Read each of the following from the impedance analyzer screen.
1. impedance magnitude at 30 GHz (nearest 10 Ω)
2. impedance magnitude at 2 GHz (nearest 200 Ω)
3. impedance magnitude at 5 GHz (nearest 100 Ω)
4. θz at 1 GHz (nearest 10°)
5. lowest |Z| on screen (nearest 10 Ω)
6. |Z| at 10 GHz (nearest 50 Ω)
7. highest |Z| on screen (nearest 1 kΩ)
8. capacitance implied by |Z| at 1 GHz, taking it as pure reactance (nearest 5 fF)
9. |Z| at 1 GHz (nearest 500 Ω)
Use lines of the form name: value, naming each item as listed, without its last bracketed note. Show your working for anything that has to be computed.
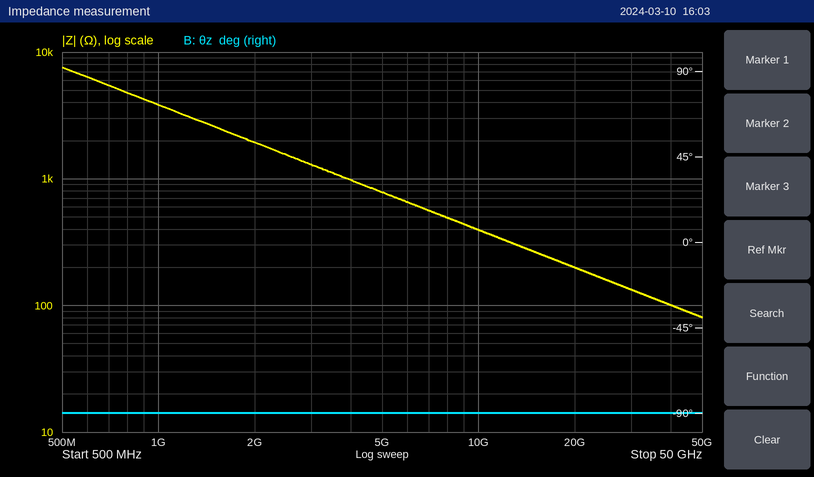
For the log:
impedance magnitude at 30 GHz: 130 Ω
impedance magnitude at 2 GHz: 2.0 kΩ
impedance magnitude at 5 GHz: 800 Ω
θz at 1 GHz: -90°
lowest |Z| on screen: 80 Ω
|Z| at 10 GHz: 400 Ω
highest |Z| on screen: 8 kΩ
capacitance implied by |Z| at 1 GHz, taking it as pure reactance: C = 1/(2π × 1 GHz × 4.0 kΩ) ≈ 40 fF
|Z| at 1 GHz: 4.0 kΩ
